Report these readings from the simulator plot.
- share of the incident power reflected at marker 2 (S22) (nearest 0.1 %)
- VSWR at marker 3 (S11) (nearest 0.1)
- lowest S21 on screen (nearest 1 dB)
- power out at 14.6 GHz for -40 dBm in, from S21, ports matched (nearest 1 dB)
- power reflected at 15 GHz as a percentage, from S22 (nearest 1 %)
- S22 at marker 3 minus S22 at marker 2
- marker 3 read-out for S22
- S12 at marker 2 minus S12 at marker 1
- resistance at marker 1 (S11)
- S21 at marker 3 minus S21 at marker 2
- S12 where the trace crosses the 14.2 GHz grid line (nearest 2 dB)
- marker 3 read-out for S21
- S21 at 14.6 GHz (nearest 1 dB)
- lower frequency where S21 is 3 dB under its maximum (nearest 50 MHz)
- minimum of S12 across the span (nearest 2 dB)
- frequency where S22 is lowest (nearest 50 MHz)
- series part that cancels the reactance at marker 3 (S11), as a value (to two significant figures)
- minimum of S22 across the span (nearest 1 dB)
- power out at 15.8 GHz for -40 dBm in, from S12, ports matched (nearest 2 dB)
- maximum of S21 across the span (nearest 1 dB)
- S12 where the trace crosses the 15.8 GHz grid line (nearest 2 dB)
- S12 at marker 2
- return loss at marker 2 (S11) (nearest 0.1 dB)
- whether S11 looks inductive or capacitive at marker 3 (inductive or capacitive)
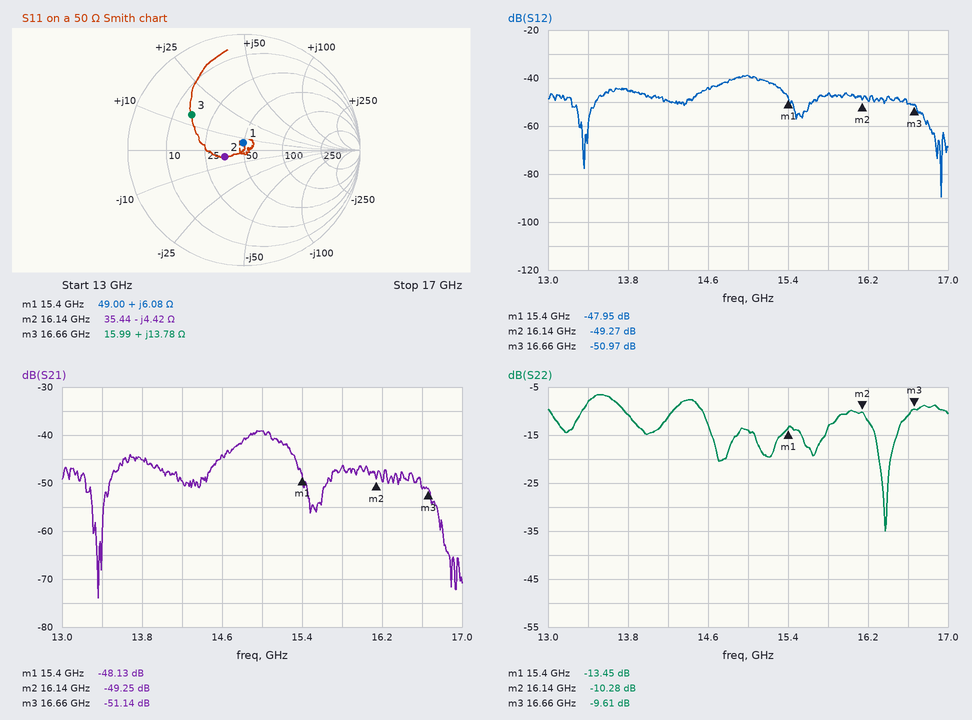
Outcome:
9.4 %
3.4
-74 dB
-84 dBm
4 %
0.67 dB
-9.61 dB
-1.32 dB
49.00 Ω
-1.89 dB
-50 dB
-51.14 dB
-44 dB
14.75 GHz
-90 dB
16.35 GHz
690 fF
-35 dB
-86 dBm
-39 dB
-46 dB
-49.27 dB
15.0 dB
inductive
